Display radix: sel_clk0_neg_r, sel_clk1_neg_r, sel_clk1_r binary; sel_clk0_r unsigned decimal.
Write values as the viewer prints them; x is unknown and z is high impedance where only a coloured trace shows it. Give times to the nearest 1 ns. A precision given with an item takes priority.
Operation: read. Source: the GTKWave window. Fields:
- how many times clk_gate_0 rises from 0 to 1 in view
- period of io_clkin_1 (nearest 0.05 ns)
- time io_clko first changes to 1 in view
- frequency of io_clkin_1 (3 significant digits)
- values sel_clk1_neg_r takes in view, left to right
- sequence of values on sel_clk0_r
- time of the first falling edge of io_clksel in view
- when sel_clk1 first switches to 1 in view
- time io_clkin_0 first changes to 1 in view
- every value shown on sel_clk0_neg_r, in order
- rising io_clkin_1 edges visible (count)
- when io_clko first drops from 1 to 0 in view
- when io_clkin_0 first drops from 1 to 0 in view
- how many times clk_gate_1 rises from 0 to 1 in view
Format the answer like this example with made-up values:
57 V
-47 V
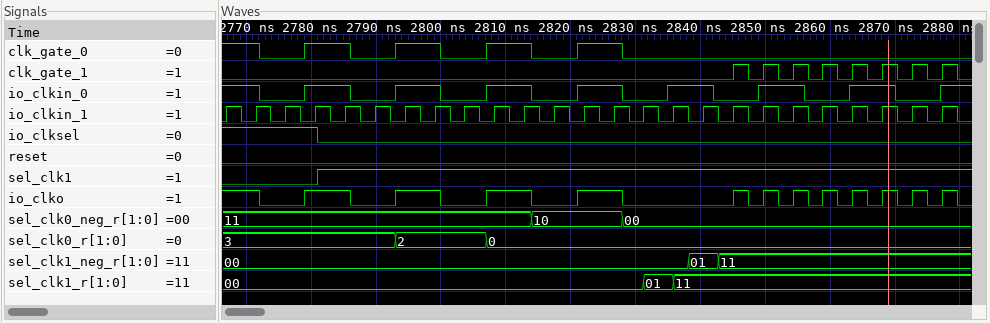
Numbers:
4
4.6 ns
2779 ns
217 MHz
00, 01, 11
3, 2, 0
2781 ns
2781 ns
2779 ns
11, 10, 00
25
2772 ns
2772 ns
8
